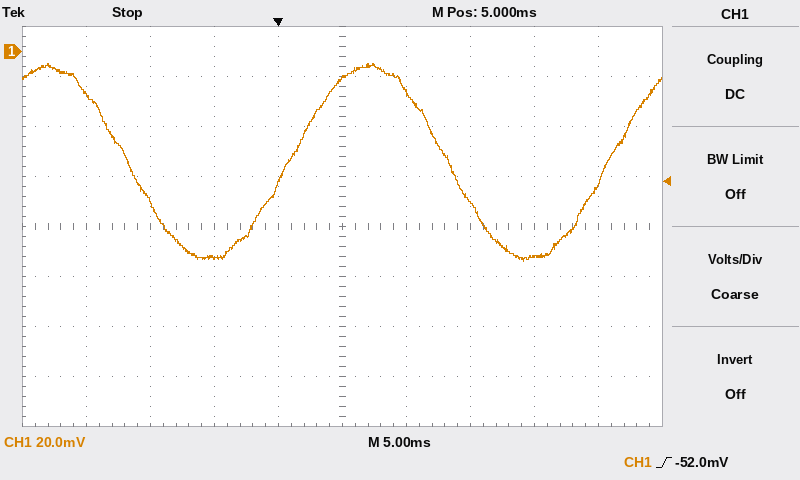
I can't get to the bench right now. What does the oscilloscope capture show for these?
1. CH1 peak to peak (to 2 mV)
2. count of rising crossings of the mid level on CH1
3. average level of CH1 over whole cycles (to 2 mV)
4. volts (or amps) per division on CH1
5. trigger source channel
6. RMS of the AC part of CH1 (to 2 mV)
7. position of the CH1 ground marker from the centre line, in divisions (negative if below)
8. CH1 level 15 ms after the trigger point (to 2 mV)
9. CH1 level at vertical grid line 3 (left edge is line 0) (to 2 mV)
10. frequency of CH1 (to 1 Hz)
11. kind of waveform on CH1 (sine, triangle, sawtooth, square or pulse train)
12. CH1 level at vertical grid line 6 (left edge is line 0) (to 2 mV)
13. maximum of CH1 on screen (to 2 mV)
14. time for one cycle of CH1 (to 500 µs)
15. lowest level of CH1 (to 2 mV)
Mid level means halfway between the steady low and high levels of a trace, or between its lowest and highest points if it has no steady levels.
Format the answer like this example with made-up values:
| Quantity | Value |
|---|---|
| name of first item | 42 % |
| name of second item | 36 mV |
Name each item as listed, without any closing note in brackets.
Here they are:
| Quantity | Value |
|---|---|
| CH1 peak to peak | 80 mV |
| count of rising crossings of the mid level on CH1 | 2 |
| average level of CH1 over whole cycles | -44 mV |
| volts (or amps) per division on CH1 | 20 mV |
| trigger source channel | CH1 |
| RMS of the AC part of CH1 | 28 mV |
| position of the CH1 ground marker from the centre line, in divisions | +3.5 div |
| CH1 level 15 ms after the trigger point | -60 mV |
| CH1 level at vertical grid line 3 (left edge is line 0) | -82 mV |
| frequency of CH1 | 40 Hz |
| kind of waveform on CH1 | sine |
| CH1 level at vertical grid line 6 (left edge is line 0) | -16 mV |
| maximum of CH1 on screen | -4 mV |
| time for one cycle of CH1 | 25.0 ms |
| lowest level of CH1 | -84 mV |
